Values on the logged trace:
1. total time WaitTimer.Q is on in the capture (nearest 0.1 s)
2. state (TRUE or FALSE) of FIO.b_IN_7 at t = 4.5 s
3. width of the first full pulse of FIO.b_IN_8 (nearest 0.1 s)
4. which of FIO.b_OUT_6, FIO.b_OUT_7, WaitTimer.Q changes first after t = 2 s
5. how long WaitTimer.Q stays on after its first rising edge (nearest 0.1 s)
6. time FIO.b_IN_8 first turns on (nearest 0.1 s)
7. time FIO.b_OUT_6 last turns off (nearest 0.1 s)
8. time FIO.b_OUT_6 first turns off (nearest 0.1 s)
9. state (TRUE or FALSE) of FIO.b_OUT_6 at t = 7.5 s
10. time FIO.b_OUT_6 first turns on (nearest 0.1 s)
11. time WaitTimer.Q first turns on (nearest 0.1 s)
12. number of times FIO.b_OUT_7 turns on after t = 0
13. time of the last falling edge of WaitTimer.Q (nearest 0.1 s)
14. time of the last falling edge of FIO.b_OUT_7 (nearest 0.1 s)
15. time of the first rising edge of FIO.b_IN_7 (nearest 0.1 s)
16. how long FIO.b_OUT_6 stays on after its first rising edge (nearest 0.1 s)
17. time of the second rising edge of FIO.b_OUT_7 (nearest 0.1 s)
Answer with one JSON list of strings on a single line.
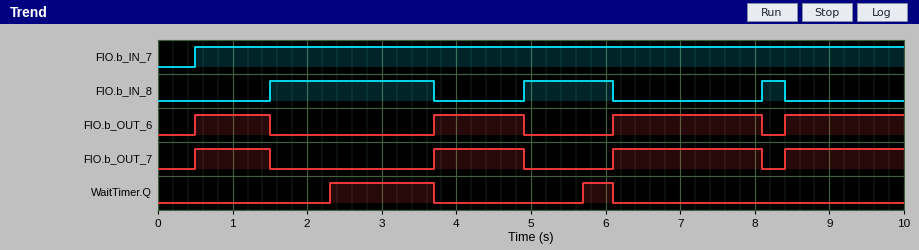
["1.8 s", "TRUE", "2.2 s", "WaitTimer.Q", "1.4 s", "1.5 s", "8.1 s", "1.5 s", "TRUE", "0.5 s", "2.3 s", "4", "6.1 s", "8.1 s", "0.5 s", "1.0 s", "3.7 s"]
